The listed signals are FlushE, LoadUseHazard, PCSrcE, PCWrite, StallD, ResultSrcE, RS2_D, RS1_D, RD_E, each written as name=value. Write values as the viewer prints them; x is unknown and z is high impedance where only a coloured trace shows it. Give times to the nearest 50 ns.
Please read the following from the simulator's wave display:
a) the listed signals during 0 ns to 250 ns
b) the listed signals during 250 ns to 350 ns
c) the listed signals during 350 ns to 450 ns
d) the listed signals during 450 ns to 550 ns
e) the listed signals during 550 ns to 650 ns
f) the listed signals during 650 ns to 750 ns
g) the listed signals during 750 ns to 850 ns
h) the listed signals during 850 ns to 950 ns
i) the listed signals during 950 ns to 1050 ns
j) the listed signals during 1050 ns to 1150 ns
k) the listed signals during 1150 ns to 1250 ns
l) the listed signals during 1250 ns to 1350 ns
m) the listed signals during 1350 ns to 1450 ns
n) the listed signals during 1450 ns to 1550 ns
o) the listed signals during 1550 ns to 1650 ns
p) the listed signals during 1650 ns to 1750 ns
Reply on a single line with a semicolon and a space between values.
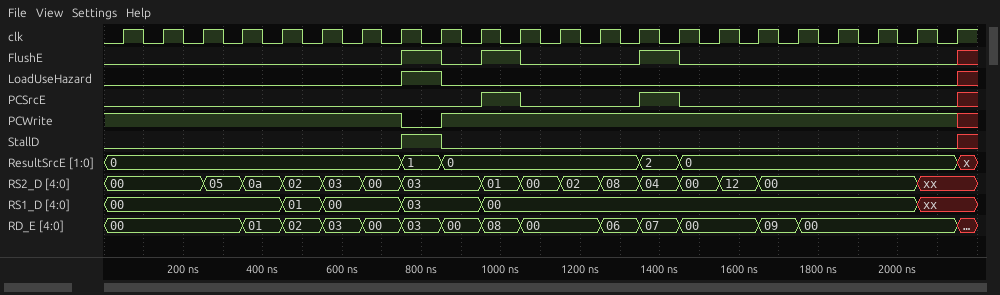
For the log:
FlushE=0, LoadUseHazard=0, PCSrcE=0, PCWrite=1, StallD=0, ResultSrcE=0, RS2_D=00, RS1_D=00, RD_E=00; FlushE=0, LoadUseHazard=0, PCSrcE=0, PCWrite=1, StallD=0, ResultSrcE=0, RS2_D=05, RS1_D=00, RD_E=00; FlushE=0, LoadUseHazard=0, PCSrcE=0, PCWrite=1, StallD=0, ResultSrcE=0, RS2_D=0a, RS1_D=00, RD_E=01; FlushE=0, LoadUseHazard=0, PCSrcE=0, PCWrite=1, StallD=0, ResultSrcE=0, RS2_D=02, RS1_D=01, RD_E=02; FlushE=0, LoadUseHazard=0, PCSrcE=0, PCWrite=1, StallD=0, ResultSrcE=0, RS2_D=03, RS1_D=00, RD_E=03; FlushE=0, LoadUseHazard=0, PCSrcE=0, PCWrite=1, StallD=0, ResultSrcE=0, RS2_D=00, RS1_D=00, RD_E=00; FlushE=1, LoadUseHazard=1, PCSrcE=0, PCWrite=0, StallD=1, ResultSrcE=1, RS2_D=03, RS1_D=03, RD_E=03; FlushE=0, LoadUseHazard=0, PCSrcE=0, PCWrite=1, StallD=0, ResultSrcE=0, RS2_D=03, RS1_D=03, RD_E=00; FlushE=1, LoadUseHazard=0, PCSrcE=1, PCWrite=1, StallD=0, ResultSrcE=0, RS2_D=01, RS1_D=00, RD_E=08; FlushE=0, LoadUseHazard=0, PCSrcE=0, PCWrite=1, StallD=0, ResultSrcE=0, RS2_D=00, RS1_D=00, RD_E=00; FlushE=0, LoadUseHazard=0, PCSrcE=0, PCWrite=1, StallD=0, ResultSrcE=0, RS2_D=02, RS1_D=00, RD_E=00; FlushE=0, LoadUseHazard=0, PCSrcE=0, PCWrite=1, StallD=0, ResultSrcE=0, RS2_D=08, RS1_D=00, RD_E=06; FlushE=1, LoadUseHazard=0, PCSrcE=1, PCWrite=1, StallD=0, ResultSrcE=2, RS2_D=04, RS1_D=00, RD_E=07; FlushE=0, LoadUseHazard=0, PCSrcE=0, PCWrite=1, StallD=0, ResultSrcE=0, RS2_D=00, RS1_D=00, RD_E=00; FlushE=0, LoadUseHazard=0, PCSrcE=0, PCWrite=1, StallD=0, ResultSrcE=0, RS2_D=12, RS1_D=00, RD_E=00; FlushE=0, LoadUseHazard=0, PCSrcE=0, PCWrite=1, StallD=0, ResultSrcE=0, RS2_D=00, RS1_D=00, RD_E=09
